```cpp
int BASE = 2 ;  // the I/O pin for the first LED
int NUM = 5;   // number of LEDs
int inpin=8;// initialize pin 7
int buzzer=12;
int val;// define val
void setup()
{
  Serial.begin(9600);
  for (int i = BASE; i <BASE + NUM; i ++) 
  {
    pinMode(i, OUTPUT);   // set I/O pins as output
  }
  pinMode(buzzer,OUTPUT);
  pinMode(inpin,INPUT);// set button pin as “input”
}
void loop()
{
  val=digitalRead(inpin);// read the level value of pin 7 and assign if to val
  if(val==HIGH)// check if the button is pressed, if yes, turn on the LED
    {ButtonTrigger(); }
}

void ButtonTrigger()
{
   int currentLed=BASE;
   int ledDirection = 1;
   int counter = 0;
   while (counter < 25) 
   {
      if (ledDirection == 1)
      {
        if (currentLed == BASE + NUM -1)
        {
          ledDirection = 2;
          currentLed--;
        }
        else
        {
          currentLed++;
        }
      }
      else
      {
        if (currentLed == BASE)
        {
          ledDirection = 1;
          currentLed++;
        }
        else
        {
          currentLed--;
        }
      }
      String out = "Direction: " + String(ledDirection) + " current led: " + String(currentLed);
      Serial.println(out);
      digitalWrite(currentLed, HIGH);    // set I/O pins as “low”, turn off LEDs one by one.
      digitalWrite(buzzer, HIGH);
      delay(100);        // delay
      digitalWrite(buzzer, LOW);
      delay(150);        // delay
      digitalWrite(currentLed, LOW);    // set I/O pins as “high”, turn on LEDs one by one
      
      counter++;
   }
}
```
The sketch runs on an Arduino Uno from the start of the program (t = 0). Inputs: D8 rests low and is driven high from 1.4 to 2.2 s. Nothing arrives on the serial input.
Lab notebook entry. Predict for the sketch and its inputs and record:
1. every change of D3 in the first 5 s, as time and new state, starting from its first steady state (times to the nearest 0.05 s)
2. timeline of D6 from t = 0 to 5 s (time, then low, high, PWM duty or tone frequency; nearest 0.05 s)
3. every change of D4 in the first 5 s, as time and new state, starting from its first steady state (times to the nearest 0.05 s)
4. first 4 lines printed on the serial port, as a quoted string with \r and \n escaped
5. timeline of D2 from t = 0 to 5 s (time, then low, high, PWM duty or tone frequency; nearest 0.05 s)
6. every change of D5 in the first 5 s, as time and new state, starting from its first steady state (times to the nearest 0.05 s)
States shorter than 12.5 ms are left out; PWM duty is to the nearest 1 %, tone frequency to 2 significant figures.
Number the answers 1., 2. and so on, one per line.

1. 0 s low; 1.4 s high; 1.65 s low; 2.9 s high; 3.15 s low; 3.4 s high; 3.65 s low; 4.9 s high
2. 0 s low; 2.15 s high; 2.4 s low; 4.15 s high; 4.4 s low
3. 0 s low; 1.65 s high; 1.9 s low; 2.65 s high; 2.9 s low; 3.65 s high; 3.9 s low; 4.65 s high; 4.9 s low
4. "Direction: 1 current led: 3\r\nDirection: 1 current led: 4\r\nDirection: 1 current led: 5\r\nDirection: 1 current led: 6\r\n"
5. 0 s low; 3.15 s high; 3.4 s low
6. 0 s low; 1.9 s high; 2.15 s low; 2.4 s high; 2.65 s low; 3.9 s high; 4.15 s low; 4.4 s high; 4.65 s low
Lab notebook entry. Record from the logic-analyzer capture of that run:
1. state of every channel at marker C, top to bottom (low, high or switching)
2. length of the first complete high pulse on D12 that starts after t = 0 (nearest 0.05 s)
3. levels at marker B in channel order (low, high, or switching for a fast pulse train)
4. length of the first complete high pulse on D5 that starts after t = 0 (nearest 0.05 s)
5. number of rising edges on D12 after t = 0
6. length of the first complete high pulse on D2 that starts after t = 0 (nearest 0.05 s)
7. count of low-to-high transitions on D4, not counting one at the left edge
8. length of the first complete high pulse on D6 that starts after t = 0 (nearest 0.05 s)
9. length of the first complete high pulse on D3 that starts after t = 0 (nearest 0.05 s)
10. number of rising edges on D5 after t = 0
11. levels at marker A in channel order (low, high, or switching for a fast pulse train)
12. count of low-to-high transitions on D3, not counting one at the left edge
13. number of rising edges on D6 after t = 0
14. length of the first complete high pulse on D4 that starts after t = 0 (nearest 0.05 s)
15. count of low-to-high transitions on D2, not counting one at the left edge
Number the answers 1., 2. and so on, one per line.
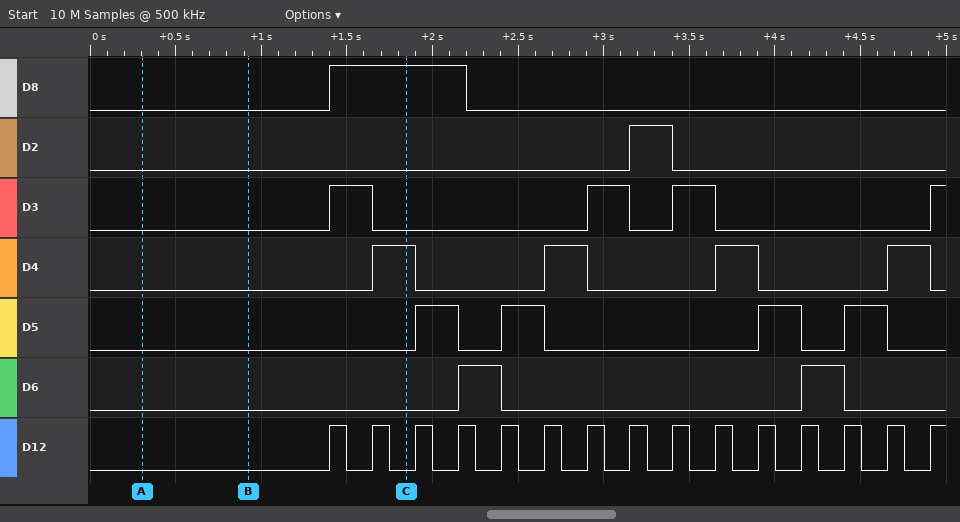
1. D8 high, D2 low, D3 low, D4 high, D5 low, D6 low, D12 low
2. 0.10 s
3. D8 low, D2 low, D3 low, D4 low, D5 low, D6 low, D12 low
4. 0.25 s
5. 15
6. 0.25 s
7. 4
8. 0.25 s
9. 0.25 s
10. 4
11. D8 low, D2 low, D3 low, D4 low, D5 low, D6 low, D12 low
12. 4
13. 2
14. 0.25 s
15. 1
